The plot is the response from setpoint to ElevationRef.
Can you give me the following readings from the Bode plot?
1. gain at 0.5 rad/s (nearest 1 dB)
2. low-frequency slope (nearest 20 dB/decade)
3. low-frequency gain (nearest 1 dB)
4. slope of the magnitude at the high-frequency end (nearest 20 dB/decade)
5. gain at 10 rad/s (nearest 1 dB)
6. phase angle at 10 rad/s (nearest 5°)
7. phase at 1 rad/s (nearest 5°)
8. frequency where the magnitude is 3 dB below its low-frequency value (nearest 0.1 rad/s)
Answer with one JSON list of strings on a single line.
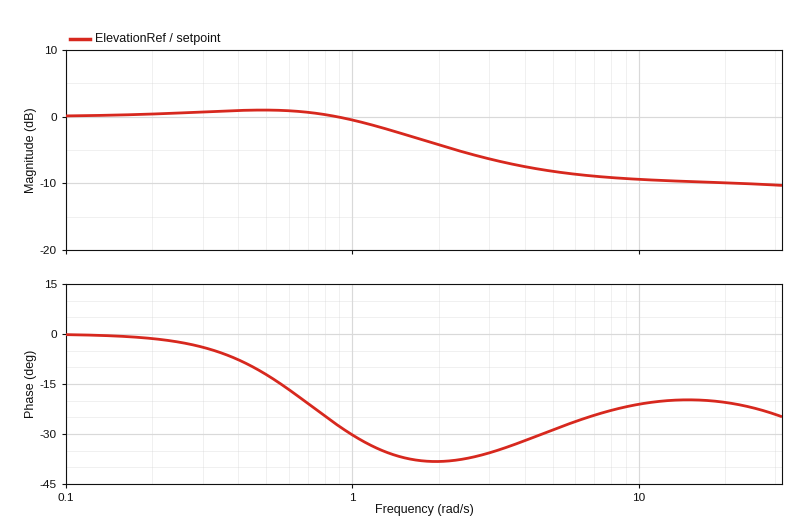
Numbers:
["1 dB", "0 dB/decade", "0 dB", "0 dB/decade", "-9 dB", "-20°", "-30°", "1.6 rad/s"]
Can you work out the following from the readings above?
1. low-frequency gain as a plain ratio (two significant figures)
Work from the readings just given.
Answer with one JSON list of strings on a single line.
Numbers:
["1.0"]
